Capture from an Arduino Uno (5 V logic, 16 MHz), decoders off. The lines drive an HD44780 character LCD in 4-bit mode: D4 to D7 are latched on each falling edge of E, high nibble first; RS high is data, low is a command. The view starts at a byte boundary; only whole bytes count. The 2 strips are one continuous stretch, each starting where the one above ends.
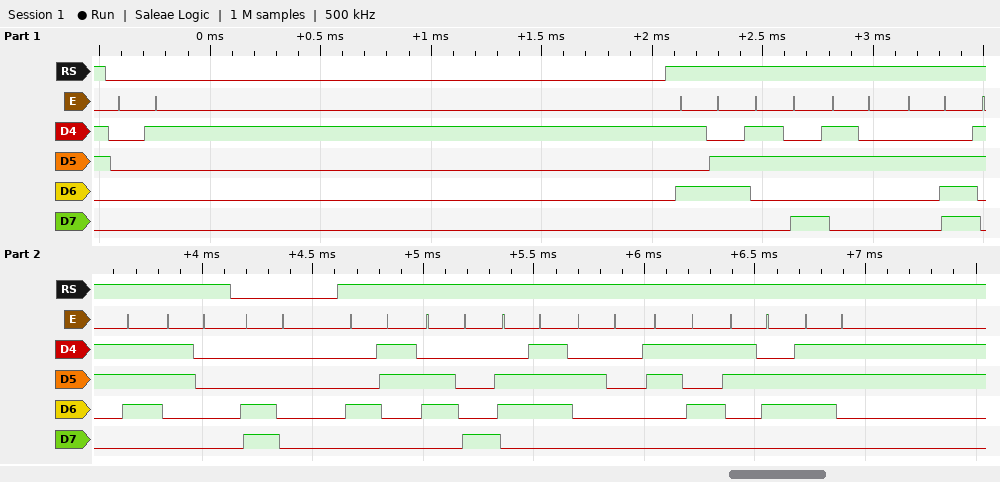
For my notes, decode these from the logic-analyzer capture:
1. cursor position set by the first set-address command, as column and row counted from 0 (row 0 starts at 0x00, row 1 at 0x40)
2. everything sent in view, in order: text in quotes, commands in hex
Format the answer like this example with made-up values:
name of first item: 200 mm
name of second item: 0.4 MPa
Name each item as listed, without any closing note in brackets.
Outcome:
cursor position set by the first set-address command, as column and row counted from 0: column 0, row 1
everything sent in view, in order: text in quotes, commands in hex: 0x01 "V:2.70" 0xC0 "Chg 56s"
